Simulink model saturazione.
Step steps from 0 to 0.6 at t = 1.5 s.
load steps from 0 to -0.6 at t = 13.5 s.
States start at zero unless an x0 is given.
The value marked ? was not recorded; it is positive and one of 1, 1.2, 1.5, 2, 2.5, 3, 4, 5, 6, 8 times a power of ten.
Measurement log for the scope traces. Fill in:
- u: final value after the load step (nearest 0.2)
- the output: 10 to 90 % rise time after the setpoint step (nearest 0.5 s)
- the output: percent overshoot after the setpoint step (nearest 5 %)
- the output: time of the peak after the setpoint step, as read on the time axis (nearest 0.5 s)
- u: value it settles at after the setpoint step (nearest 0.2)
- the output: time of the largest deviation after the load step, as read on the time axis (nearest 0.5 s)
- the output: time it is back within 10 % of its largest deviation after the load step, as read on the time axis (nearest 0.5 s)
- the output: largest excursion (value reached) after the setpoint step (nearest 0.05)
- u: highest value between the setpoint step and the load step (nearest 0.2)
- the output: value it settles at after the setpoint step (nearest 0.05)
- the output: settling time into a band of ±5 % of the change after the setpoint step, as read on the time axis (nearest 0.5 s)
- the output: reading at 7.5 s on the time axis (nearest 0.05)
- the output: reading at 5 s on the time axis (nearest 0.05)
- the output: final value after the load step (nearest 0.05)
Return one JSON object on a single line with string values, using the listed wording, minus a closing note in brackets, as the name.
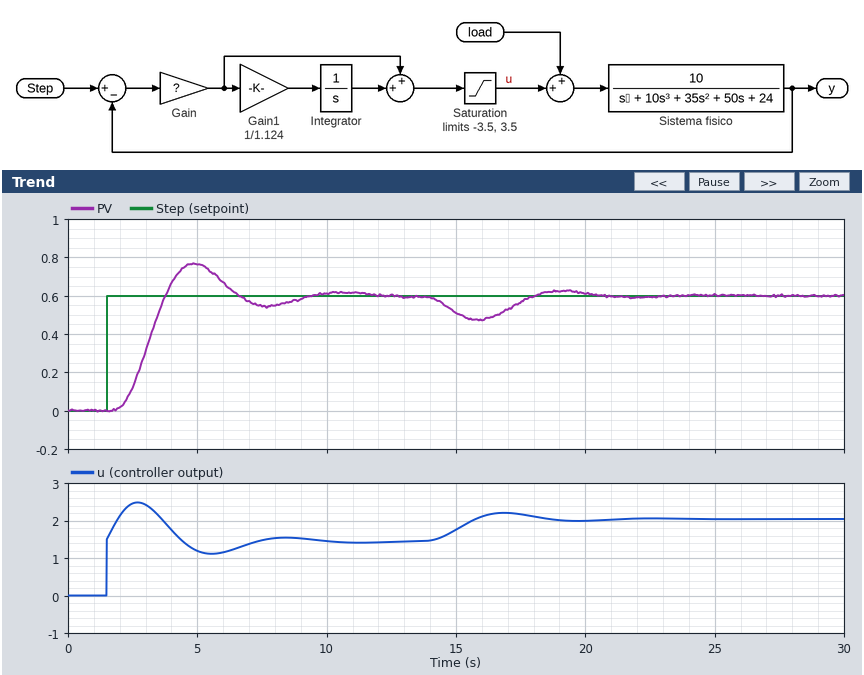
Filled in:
{"u: final value after the load step": "2.0", "the output: 10 to 90 % rise time after the setpoint step": "1.5 s", "the output: percent overshoot after the setpoint step": "30 %", "the output: time of the peak after the setpoint step, as read on the time axis": "5.0 s", "u: value it settles at after the setpoint step": "1.4", "the output: time of the largest deviation after the load step, as read on the time axis": "16.0 s", "the output: time it is back within 10 % of its largest deviation after the load step, as read on the time axis": "20.0 s", "the output: largest excursion (value reached) after the setpoint step": "0.75", "u: highest value between the setpoint step and the load step": "2.4", "the output: value it settles at after the setpoint step": "0.60", "the output: settling time into a band of ±5 % of the change after the setpoint step, as read on the time axis": "8.5 s", "the output: reading at 7.5 s on the time axis": "0.55", "the output: reading at 5 s on the time axis": "0.75", "the output: final value after the load step": "0.60"}
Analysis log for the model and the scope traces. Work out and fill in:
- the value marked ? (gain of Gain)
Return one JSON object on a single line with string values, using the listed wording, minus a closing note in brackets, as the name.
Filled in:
{"the value marked ?": "2.5"}
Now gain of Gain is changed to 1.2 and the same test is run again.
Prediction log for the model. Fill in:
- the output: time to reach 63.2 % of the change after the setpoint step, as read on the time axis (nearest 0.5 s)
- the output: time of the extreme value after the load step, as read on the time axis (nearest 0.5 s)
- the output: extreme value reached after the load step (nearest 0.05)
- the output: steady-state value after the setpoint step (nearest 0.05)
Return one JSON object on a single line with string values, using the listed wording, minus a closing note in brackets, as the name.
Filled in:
{"the output: time to reach 63.2 % of the change after the setpoint step, as read on the time axis": "4.0 s", "the output: time of the extreme value after the load step, as read on the time axis": "16.5 s", "the output: extreme value reached after the load step": "0.45", "the output: steady-state value after the setpoint step": "0.60"}
